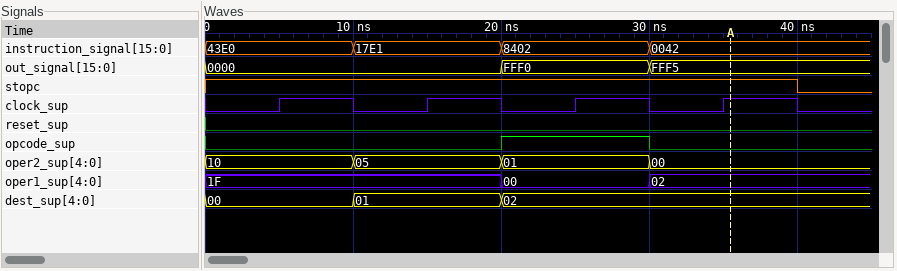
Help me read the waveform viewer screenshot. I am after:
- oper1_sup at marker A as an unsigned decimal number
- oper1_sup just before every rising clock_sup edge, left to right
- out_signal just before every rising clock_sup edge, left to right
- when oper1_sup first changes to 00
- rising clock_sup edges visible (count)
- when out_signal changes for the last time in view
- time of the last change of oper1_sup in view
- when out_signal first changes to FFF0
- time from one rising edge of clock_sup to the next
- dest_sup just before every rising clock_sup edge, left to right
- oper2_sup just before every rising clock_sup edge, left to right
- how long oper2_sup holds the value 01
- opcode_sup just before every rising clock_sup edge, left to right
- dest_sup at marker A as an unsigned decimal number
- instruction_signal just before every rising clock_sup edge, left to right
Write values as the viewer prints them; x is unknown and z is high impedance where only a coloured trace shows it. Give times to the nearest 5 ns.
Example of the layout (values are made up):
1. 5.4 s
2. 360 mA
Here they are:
1. 2
2. 1F, 1F, 00, 02
3. 0000, 0000, FFF0, FFF5
4. 20 ns
5. 4
6. 30 ns
7. 30 ns
8. 20 ns
9. 10 ns
10. 00, 01, 02, 02
11. 10, 05, 01, 00
12. 10 ns
13. 0 0 1 0
14. 2
15. 43E0, 17E1, 8402, 0042
